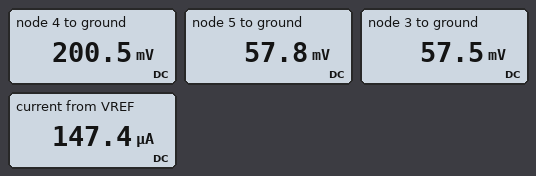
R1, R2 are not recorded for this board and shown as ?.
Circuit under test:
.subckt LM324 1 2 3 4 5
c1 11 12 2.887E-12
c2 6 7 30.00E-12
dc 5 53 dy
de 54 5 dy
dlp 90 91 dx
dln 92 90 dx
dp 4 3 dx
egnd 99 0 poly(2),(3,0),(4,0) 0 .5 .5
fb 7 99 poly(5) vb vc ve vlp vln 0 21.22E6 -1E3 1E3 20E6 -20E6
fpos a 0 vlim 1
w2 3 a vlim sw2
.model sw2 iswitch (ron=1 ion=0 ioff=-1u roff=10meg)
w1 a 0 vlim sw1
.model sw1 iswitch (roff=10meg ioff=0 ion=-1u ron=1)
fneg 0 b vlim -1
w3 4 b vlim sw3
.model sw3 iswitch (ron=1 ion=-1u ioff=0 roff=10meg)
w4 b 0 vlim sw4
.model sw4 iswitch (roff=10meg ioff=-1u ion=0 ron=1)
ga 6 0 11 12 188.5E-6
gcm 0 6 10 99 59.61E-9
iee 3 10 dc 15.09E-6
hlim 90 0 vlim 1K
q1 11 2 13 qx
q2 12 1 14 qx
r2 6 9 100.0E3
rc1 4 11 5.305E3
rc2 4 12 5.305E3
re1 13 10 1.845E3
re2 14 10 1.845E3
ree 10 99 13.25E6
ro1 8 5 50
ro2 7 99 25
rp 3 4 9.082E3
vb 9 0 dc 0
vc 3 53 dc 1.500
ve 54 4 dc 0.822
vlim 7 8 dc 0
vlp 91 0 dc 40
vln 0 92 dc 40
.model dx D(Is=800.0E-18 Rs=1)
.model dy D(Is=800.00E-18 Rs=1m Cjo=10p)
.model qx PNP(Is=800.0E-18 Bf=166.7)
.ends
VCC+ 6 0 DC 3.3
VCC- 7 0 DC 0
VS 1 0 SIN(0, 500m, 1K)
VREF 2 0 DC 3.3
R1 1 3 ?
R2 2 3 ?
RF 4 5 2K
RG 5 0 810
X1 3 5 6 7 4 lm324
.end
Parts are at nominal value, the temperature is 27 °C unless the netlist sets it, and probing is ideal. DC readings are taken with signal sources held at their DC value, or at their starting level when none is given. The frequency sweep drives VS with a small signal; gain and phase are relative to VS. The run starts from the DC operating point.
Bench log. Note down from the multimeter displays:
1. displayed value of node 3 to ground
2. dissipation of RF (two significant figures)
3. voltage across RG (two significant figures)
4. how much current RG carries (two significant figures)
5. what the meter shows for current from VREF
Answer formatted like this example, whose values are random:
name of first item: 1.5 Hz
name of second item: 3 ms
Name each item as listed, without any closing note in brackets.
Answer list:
displayed value of node 3 to ground: 57.5 mV
dissipation of RF: 10 µW
voltage across RG: 58 mV
how much current RG carries: 71 µA
what the meter shows for current from VREF: 147.4 µA
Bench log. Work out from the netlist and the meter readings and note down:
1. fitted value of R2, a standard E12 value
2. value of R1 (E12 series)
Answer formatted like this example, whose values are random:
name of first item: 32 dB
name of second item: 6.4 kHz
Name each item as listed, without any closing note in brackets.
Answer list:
fitted value of R2, a standard E12 value: 22 kΩ
value of R1: 390 Ω
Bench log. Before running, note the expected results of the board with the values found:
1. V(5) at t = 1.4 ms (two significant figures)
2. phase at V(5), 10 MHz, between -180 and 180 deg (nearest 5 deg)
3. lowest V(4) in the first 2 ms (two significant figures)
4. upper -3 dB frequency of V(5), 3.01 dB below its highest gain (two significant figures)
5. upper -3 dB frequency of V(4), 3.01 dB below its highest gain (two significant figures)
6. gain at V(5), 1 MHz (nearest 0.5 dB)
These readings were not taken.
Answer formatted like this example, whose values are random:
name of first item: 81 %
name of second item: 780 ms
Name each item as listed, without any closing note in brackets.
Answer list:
V(5) at t = 1.4 ms: 350 mV
phase at V(5), 10 MHz, between -180 and 180 deg: -155 deg
lowest V(4) in the first 2 ms: 5.7 mV
upper -3 dB frequency of V(5), 3.01 dB below its highest gain: 290 kHz
upper -3 dB frequency of V(4), 3.01 dB below its highest gain: 290 kHz
gain at V(5), 1 MHz: -11.5 dB
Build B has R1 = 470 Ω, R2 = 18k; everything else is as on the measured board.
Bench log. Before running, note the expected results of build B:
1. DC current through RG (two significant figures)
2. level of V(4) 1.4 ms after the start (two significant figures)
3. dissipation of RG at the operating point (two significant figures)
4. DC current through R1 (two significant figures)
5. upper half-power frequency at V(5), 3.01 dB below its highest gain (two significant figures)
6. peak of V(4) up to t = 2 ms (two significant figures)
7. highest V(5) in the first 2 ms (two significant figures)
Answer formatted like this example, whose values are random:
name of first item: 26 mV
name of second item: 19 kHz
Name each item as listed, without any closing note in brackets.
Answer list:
DC current through RG: 100 µA
level of V(4) 1.4 ms after the start: 1.3 V
dissipation of RG at the operating point: 8.8 µW
DC current through R1: 180 µA
upper half-power frequency at V(5), 3.01 dB below its highest gain: 300 kHz
peak of V(4) up to t = 2 ms: 2.0 V
highest V(5) in the first 2 ms: 570 mV
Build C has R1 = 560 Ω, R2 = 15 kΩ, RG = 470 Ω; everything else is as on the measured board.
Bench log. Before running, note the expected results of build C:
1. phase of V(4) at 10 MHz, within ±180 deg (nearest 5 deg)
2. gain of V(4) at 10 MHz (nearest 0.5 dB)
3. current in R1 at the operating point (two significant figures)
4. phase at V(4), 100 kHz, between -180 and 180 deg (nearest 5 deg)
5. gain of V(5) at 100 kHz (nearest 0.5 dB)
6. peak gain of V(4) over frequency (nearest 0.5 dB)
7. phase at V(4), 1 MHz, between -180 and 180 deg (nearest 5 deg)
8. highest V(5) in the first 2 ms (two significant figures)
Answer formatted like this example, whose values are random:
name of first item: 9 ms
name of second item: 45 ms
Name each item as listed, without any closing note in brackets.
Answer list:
phase of V(4) at 10 MHz, within ±180 deg: -155 deg
gain of V(4) at 10 MHz: -27.0 dB
current in R1 at the operating point: 210 µA
phase at V(4), 100 kHz, between -180 and 180 deg: -30 deg
gain of V(5) at 100 kHz: -1.5 dB
peak gain of V(4) over frequency: 14.0 dB
phase at V(4), 1 MHz, between -180 and 180 deg: -90 deg
highest V(5) in the first 2 ms: 500 mV
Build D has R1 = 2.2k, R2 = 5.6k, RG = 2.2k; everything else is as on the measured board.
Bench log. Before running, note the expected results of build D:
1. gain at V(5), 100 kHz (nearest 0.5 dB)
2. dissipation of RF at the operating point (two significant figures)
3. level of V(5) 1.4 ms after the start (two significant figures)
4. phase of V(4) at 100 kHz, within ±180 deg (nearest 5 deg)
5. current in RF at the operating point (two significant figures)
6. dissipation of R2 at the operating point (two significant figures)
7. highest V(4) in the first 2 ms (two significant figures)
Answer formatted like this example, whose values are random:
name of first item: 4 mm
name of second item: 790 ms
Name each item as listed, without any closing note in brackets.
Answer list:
gain at V(5), 100 kHz: -3.0 dB
dissipation of RF at the operating point: 360 µW
level of V(5) 1.4 ms after the start: 1.1 V
phase of V(4) at 100 kHz, within ±180 deg: -10 deg
current in RF at the operating point: 420 µA
dissipation of R2 at the operating point: 1.0 mW
highest V(4) in the first 2 ms: 2.5 V
